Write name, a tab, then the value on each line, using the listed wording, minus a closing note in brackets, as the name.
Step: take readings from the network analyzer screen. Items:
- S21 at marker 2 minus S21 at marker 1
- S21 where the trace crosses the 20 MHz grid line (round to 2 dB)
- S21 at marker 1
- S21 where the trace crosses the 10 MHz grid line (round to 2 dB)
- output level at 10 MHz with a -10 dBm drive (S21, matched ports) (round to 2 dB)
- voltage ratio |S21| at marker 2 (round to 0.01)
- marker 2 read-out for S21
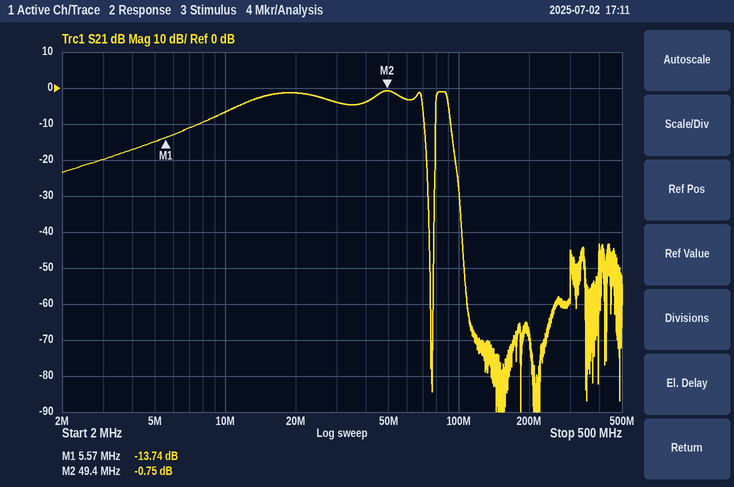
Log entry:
S21 at marker 2 minus S21 at marker 1	12.99 dB
S21 where the trace crosses the 20 MHz grid line	-2 dB
S21 at marker 1	-13.74 dB
S21 where the trace crosses the 10 MHz grid line	-6 dB
output level at 10 MHz with a -10 dBm drive (S21, matched ports)	-16 dBm
voltage ratio |S21| at marker 2	0.92
marker 2 read-out for S21	-0.75 dB
